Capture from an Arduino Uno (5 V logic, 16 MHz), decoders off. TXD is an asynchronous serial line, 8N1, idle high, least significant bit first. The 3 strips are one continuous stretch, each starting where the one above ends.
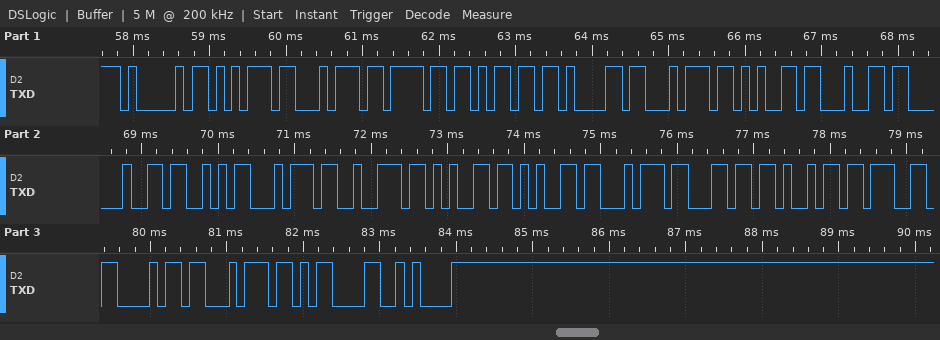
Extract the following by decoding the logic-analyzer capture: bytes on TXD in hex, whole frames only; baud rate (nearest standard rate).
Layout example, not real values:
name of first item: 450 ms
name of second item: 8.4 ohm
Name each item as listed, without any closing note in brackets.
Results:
bytes on TXD in hex, whole frames only: 0x41 0x75 0x74 0x6F 0x6D 0x61 0x74 0x65 0x64 0x20 0x53 0x74 0x72 0x65 0x65 0x74 0x6C 0x69 0x67 0x68 0x74 0x0D 0x0A
baud rate: 9600 baud
